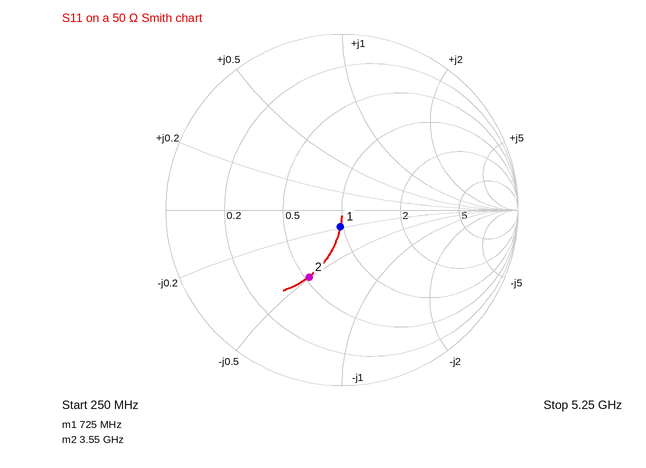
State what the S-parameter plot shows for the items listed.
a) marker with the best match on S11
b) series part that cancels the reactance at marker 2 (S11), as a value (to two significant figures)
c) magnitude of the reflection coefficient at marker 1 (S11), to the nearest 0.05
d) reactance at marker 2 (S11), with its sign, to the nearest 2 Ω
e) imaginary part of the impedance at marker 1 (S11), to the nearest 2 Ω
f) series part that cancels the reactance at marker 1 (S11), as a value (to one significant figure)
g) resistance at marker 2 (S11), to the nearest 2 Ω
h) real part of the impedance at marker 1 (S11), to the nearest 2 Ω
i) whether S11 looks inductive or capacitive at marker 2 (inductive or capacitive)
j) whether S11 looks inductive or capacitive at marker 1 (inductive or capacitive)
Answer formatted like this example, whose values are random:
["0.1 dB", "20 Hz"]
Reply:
["marker 1", "1.1 nH", "0.10", "-24 Ω", "-10 Ω", "2 nH", "26 Ω", "48 Ω", "capacitive", "capacitive"]
